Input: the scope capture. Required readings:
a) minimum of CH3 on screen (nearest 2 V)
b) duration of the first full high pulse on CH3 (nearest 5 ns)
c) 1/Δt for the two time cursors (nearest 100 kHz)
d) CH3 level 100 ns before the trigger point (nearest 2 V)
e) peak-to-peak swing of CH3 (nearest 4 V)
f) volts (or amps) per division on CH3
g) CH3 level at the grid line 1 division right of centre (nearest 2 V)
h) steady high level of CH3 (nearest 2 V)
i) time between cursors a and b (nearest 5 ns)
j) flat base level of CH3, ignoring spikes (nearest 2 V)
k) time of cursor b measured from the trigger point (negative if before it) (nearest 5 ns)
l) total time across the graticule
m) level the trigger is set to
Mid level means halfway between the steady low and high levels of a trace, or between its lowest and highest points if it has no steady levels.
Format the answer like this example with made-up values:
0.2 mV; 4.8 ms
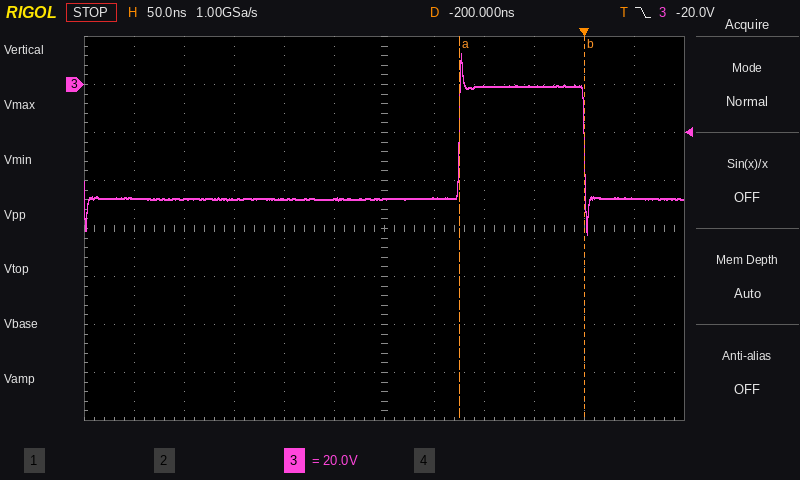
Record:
-62 V; 125 ns; 8.0 MHz; 0 V; 76 V; 20 V; -48 V; 0 V; 125 ns; -48 V; 0 ns; 600 ns; -20.0 V
